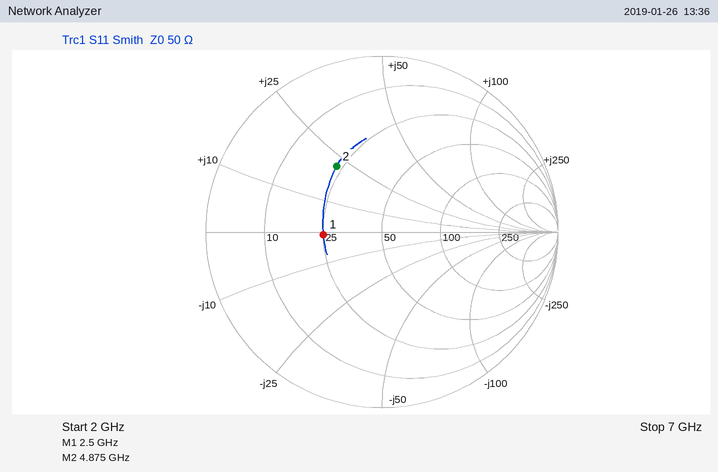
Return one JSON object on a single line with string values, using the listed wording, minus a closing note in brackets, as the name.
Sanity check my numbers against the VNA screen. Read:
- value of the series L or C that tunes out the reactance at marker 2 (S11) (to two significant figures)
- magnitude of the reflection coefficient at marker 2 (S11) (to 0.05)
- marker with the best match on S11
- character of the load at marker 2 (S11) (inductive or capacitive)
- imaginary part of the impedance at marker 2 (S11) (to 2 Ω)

{"value of the series L or C that tunes out the reactance at marker 2 (S11)": "1.5 pF", "magnitude of the reflection coefficient at marker 2 (S11)": "0.45", "marker with the best match on S11": "marker 1", "character of the load at marker 2 (S11)": "inductive", "imaginary part of the impedance at marker 2 (S11)": "+22 Ω"}
